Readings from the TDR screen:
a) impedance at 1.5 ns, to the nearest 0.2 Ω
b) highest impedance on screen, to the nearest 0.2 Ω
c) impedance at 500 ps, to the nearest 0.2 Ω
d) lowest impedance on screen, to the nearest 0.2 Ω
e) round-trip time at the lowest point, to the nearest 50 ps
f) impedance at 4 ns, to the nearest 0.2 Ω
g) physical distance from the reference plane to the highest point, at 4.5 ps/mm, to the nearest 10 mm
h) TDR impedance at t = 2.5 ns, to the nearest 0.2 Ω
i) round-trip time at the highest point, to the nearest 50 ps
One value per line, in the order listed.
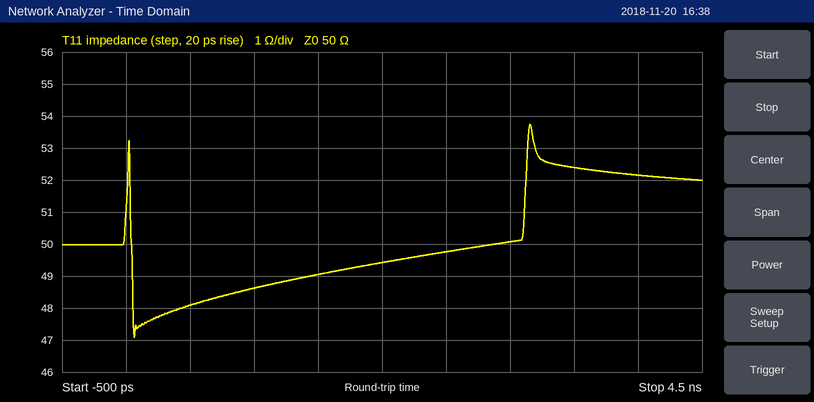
49.0 Ω
53.8 Ω
48.0 Ω
47.0 Ω
50 ps
52.2 Ω
350 mm
49.8 Ω
3.15 ns
